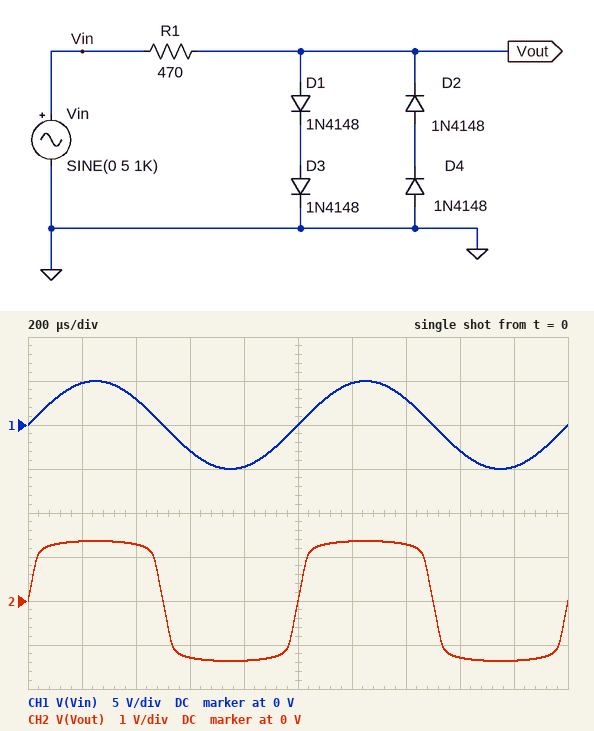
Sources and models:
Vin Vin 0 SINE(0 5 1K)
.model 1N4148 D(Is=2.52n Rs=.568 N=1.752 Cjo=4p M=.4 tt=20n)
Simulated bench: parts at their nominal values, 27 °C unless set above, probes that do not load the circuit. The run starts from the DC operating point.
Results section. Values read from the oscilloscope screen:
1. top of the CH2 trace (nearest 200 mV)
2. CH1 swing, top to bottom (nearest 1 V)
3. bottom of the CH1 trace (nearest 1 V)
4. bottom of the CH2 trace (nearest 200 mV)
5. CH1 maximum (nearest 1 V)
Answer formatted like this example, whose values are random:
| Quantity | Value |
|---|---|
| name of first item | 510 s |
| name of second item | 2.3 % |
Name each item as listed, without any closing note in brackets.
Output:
| Quantity | Value |
|---|---|
| top of the CH2 trace | 1.4 V |
| CH1 swing, top to bottom | 10 V |
| bottom of the CH1 trace | -5 V |
| bottom of the CH2 trace | -1.4 V |
| CH1 maximum | 5 V |
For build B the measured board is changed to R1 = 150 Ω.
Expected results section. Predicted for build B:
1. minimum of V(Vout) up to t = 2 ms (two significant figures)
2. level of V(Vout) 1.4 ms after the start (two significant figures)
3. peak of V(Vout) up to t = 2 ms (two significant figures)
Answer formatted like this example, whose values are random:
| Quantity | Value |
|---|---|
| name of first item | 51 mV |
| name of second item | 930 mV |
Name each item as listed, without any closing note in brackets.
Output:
| Quantity | Value |
|---|---|
| minimum of V(Vout) up to t = 2 ms | -1.5 V |
| level of V(Vout) 1.4 ms after the start | 1.4 V |
| peak of V(Vout) up to t = 2 ms | 1.5 V |
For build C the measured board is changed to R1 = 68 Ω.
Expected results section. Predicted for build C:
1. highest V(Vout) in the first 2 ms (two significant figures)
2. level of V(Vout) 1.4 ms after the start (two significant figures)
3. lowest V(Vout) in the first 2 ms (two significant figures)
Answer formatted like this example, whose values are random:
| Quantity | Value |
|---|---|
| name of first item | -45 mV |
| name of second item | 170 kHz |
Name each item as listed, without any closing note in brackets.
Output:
| Quantity | Value |
|---|---|
| highest V(Vout) in the first 2 ms | 1.6 V |
| level of V(Vout) 1.4 ms after the start | 1.5 V |
| lowest V(Vout) in the first 2 ms | -1.6 V |
